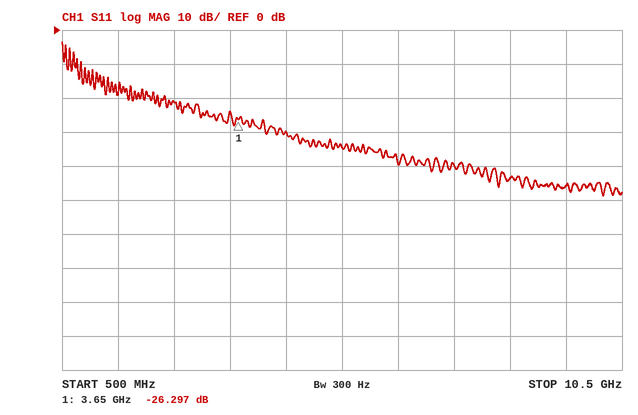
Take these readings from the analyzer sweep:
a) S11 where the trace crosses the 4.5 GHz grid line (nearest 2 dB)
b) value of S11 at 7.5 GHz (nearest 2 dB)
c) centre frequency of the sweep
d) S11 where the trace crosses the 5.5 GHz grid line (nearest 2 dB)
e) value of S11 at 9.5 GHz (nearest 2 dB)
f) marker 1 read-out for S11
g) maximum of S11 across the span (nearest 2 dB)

-30 dB
-40 dB
5.5 GHz
-34 dB
-46 dB
-26.297 dB
-4 dB
